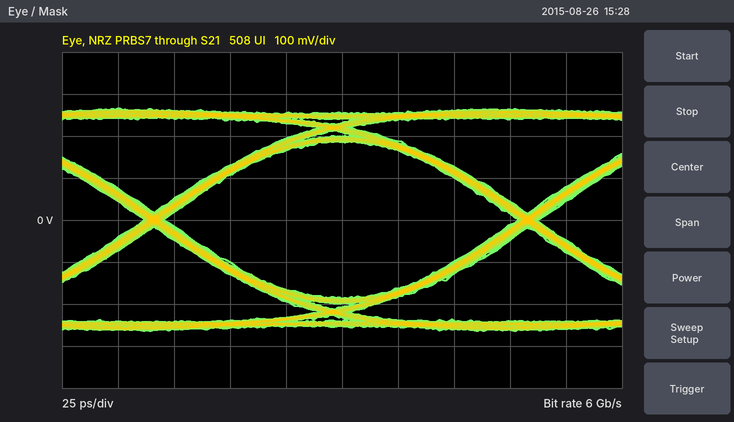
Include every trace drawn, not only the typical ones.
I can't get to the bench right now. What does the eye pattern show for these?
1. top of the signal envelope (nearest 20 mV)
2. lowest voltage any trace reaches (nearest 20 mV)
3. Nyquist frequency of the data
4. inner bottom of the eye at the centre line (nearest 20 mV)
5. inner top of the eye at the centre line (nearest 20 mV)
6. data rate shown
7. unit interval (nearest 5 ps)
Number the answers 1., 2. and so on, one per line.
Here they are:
1. 260 mV
2. -260 mV
3. 3 GHz
4. -180 mV
5. 180 mV
6. 6 Gb/s
7. 165 ps
